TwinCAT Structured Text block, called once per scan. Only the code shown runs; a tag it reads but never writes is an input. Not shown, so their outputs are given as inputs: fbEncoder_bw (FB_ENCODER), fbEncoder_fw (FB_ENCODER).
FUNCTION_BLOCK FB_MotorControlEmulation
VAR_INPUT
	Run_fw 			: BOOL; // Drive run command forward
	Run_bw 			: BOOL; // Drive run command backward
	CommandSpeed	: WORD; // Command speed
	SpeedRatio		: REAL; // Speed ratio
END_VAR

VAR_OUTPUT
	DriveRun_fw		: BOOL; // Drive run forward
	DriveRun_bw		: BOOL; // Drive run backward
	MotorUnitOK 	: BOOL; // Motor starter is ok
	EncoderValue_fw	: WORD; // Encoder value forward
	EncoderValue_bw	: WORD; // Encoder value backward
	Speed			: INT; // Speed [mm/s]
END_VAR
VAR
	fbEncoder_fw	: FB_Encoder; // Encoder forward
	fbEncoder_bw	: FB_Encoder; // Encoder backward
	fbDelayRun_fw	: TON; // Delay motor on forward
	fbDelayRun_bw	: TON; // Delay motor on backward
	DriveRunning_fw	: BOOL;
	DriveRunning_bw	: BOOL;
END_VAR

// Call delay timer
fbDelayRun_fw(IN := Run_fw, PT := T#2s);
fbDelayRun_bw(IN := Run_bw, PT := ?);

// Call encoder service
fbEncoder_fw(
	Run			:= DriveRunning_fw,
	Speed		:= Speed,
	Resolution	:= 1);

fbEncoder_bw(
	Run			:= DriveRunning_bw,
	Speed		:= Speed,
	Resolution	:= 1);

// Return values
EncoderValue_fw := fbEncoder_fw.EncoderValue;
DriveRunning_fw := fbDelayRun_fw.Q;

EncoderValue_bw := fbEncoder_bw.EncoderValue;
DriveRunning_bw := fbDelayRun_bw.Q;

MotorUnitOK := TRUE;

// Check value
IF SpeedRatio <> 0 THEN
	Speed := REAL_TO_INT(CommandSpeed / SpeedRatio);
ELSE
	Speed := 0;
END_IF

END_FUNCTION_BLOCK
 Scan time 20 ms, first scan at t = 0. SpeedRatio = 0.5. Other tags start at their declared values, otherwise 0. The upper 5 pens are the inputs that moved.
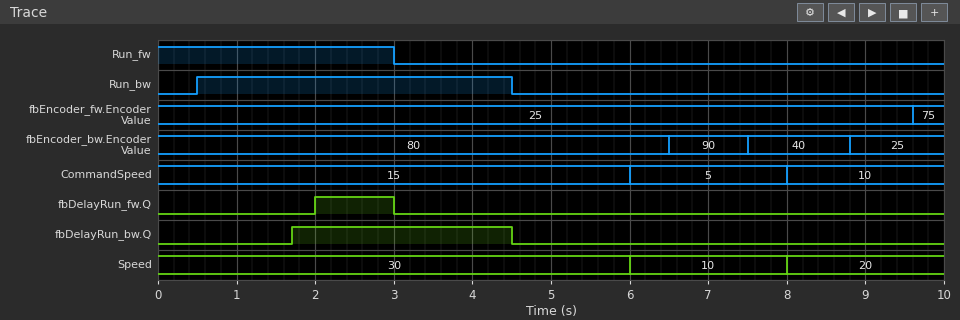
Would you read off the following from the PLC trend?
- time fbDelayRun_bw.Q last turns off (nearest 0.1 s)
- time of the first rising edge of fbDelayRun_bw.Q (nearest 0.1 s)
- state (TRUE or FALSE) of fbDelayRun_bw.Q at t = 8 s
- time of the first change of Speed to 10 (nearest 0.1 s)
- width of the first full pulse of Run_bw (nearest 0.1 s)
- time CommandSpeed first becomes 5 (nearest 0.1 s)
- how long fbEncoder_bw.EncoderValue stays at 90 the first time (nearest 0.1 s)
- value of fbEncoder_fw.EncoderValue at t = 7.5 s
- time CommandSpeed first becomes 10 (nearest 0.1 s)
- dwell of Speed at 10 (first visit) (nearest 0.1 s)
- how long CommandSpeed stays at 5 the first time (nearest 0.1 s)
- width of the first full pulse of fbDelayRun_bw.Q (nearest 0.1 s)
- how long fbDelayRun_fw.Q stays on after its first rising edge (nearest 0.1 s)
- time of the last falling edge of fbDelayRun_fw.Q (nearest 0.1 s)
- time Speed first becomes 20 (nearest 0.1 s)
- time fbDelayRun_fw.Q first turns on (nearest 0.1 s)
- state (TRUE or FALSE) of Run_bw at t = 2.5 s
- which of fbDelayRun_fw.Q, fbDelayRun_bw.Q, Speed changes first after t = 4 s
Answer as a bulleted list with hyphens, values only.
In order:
- 4.5 s
- 1.7 s
- FALSE
- 6.0 s
- 4.0 s
- 6.0 s
- 1.0 s
- 25
- 8.0 s
- 2.0 s
- 2.0 s
- 2.8 s
- 1.0 s
- 3.0 s
- 8.0 s
- 2.0 s
- TRUE
- fbDelayRun_bw.Q
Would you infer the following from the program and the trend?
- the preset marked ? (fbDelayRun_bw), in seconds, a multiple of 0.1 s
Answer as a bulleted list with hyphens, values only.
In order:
- 1.2 s
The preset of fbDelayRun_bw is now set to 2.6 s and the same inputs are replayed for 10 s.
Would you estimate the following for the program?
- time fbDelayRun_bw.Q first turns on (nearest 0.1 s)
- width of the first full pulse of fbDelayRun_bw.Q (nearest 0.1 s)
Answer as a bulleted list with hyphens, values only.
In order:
- 3.1 s
- 1.4 s
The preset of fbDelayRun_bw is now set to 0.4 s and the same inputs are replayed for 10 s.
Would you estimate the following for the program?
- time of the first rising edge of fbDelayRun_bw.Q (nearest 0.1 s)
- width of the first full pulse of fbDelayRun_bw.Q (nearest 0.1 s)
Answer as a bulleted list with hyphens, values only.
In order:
- 0.9 s
- 3.6 s
